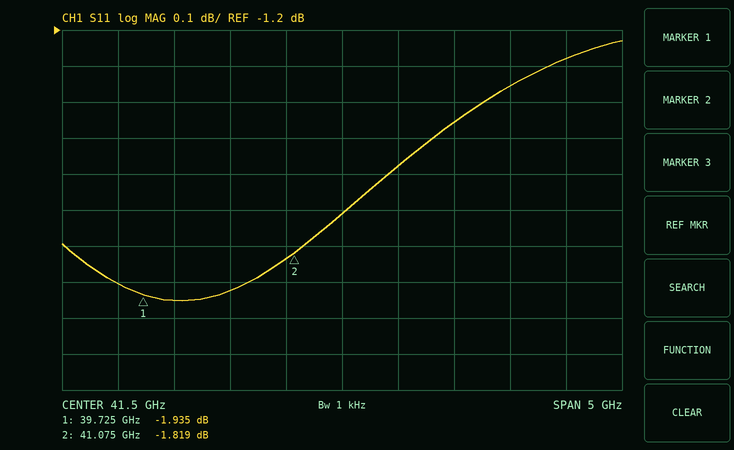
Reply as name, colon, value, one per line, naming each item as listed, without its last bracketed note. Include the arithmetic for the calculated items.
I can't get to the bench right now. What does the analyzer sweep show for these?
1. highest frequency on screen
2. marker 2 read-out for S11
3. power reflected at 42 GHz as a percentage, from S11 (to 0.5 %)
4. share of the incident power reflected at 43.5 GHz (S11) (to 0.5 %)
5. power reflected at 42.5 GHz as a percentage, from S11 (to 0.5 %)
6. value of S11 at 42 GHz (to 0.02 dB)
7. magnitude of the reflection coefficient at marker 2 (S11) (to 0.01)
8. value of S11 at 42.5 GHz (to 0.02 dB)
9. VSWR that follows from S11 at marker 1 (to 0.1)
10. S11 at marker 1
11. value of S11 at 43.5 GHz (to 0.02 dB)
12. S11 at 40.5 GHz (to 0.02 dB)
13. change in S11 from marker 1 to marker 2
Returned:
highest frequency on screen: 44 GHz
marker 2 read-out for S11: -1.819 dB
power reflected at 42 GHz as a percentage, from S11: 10^(-1.58/10) ≈ 69.5 %
share of the incident power reflected at 43.5 GHz (S11): 10^(-1.28/10) ≈ 74.5 %
power reflected at 42.5 GHz as a percentage, from S11: 10^(-1.46/10) ≈ 71.4 %, so 71.5 % to the nearest 0.5 %
value of S11 at 42 GHz: -1.58 dB
magnitude of the reflection coefficient at marker 2 (S11): 10^(-1.819/20) ≈ 0.81
value of S11 at 42.5 GHz: -1.46 dB
VSWR that follows from S11 at marker 1: (1 + 0.8003)/(1 − 0.8003) ≈ 9.0
S11 at marker 1: -1.935 dB
value of S11 at 43.5 GHz: -1.28 dB
S11 at 40.5 GHz: -1.92 dB
change in S11 from marker 1 to marker 2: -1.819 − (-1.935) = 0.116 dB
